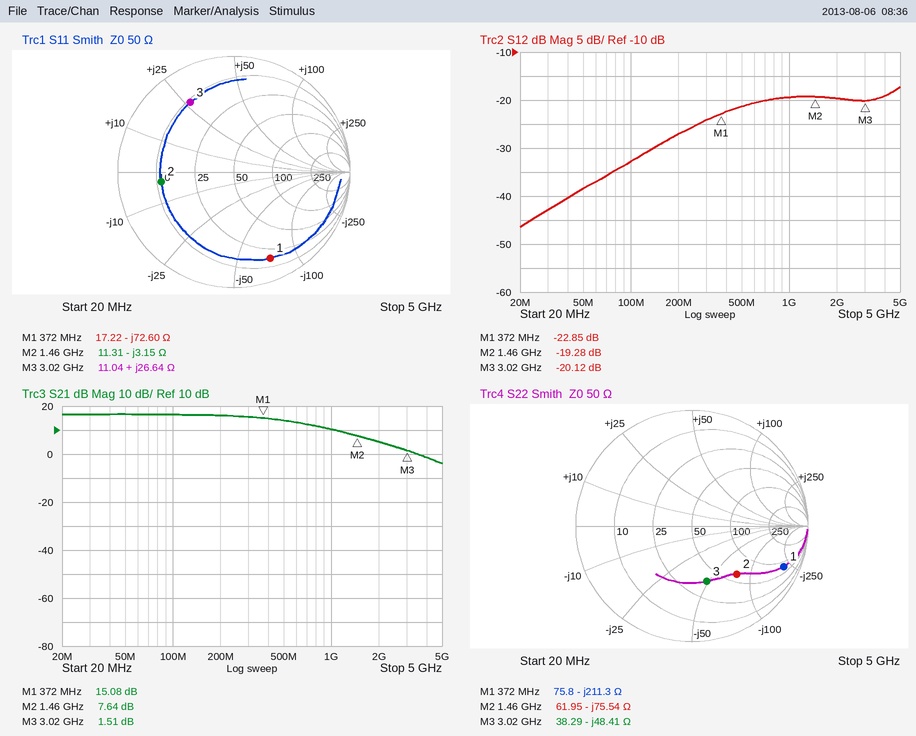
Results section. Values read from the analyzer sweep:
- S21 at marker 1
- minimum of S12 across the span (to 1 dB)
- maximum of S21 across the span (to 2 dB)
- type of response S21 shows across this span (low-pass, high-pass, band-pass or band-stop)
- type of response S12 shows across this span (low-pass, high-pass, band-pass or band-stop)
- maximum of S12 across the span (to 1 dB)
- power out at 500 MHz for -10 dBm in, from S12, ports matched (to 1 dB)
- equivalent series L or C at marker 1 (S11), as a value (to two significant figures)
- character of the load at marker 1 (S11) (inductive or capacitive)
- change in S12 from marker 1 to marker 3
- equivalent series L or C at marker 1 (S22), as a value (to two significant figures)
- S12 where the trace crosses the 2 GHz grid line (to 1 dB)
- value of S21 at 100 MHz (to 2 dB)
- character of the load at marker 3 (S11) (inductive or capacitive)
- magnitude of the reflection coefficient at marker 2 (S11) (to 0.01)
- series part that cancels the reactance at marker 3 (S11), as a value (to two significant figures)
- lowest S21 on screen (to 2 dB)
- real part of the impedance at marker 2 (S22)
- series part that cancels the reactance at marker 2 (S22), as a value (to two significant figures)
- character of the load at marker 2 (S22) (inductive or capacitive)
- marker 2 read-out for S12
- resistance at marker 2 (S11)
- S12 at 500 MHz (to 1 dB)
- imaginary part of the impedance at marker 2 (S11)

15.08 dB
-46 dB
16 dB
low-pass
high-pass
-17 dB
-31 dBm
5.9 pF
capacitive
2.73 dB
2.0 pF
-20 dB
16 dB
inductive
0.63
2.0 pF
-4 dB
61.95 Ω
8.2 nH
capacitive
-19.28 dB
11.31 Ω
-21 dB
-3.15 Ω
